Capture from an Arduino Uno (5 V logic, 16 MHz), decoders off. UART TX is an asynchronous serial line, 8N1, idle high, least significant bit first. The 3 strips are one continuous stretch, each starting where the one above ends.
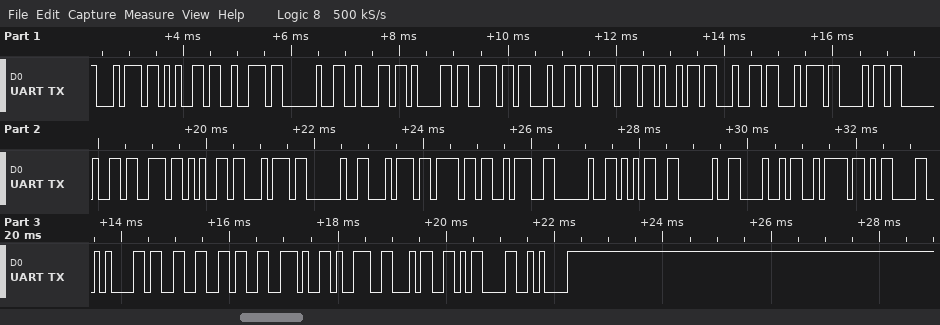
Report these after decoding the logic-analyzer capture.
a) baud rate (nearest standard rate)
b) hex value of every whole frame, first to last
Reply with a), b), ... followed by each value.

a) 9600 baud
b) 74 65 72 20 62 61 6E 64 77 69 64 74 68 20 73 65 74 20 74 6F 3A 20 35 20 48 7A 0D 0A 33 36 2E 39 34 0D 0A
